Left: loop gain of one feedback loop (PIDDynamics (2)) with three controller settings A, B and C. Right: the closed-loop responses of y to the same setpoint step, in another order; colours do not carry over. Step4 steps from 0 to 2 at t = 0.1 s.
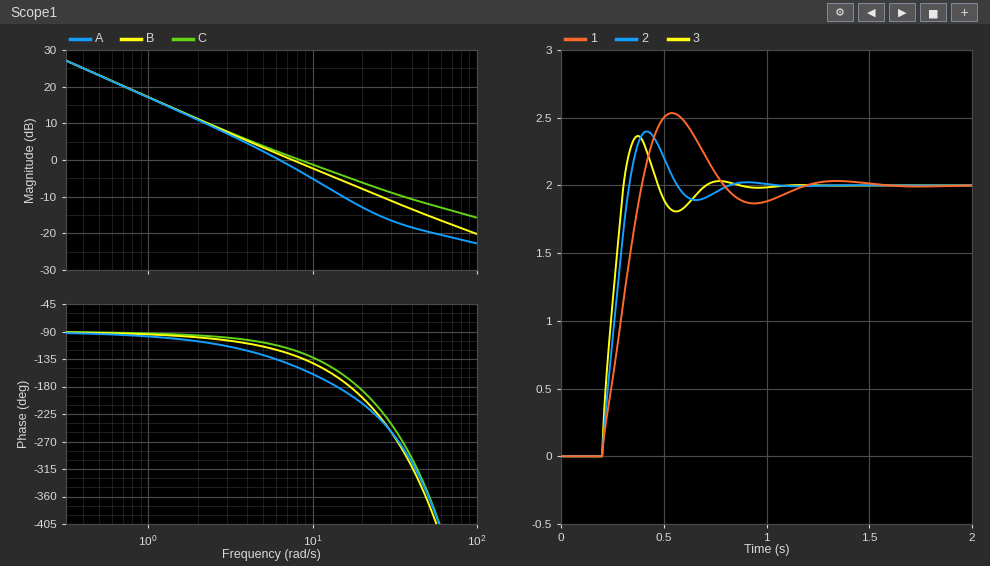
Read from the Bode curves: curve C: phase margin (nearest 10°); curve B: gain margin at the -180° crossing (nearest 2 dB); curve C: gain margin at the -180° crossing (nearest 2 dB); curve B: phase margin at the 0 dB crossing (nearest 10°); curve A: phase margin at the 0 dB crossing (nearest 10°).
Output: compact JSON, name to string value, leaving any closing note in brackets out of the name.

{"curve C: phase margin": "60°", "curve B: gain margin at the -180° crossing": "6 dB", "curve C: gain margin at the -180° crossing": "6 dB", "curve B: phase margin at the 0 dB crossing": "50°", "curve A: phase margin at the 0 dB crossing": "40°"}
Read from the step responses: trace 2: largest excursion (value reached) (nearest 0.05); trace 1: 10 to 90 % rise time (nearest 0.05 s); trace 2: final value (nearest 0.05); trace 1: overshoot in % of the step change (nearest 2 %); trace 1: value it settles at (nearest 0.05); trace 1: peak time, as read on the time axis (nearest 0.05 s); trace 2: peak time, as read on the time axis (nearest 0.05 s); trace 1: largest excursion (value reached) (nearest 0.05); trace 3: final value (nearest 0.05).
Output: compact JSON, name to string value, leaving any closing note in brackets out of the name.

{"trace 2: largest excursion (value reached)": "2.40", "trace 1: 10 to 90 % rise time": "0.15 s", "trace 2: final value": "2.00", "trace 1: overshoot in % of the step change": "26 %", "trace 1: value it settles at": "2.00", "trace 1: peak time, as read on the time axis": "0.55 s", "trace 2: peak time, as read on the time axis": "0.40 s", "trace 1: largest excursion (value reached)": "2.55", "trace 3: final value": "2.00"}
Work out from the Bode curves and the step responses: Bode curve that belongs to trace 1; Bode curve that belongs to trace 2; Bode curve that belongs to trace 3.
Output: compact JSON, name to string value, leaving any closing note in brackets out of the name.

{"Bode curve that belongs to trace 1": "A", "Bode curve that belongs to trace 2": "B", "Bode curve that belongs to trace 3": "C"}
